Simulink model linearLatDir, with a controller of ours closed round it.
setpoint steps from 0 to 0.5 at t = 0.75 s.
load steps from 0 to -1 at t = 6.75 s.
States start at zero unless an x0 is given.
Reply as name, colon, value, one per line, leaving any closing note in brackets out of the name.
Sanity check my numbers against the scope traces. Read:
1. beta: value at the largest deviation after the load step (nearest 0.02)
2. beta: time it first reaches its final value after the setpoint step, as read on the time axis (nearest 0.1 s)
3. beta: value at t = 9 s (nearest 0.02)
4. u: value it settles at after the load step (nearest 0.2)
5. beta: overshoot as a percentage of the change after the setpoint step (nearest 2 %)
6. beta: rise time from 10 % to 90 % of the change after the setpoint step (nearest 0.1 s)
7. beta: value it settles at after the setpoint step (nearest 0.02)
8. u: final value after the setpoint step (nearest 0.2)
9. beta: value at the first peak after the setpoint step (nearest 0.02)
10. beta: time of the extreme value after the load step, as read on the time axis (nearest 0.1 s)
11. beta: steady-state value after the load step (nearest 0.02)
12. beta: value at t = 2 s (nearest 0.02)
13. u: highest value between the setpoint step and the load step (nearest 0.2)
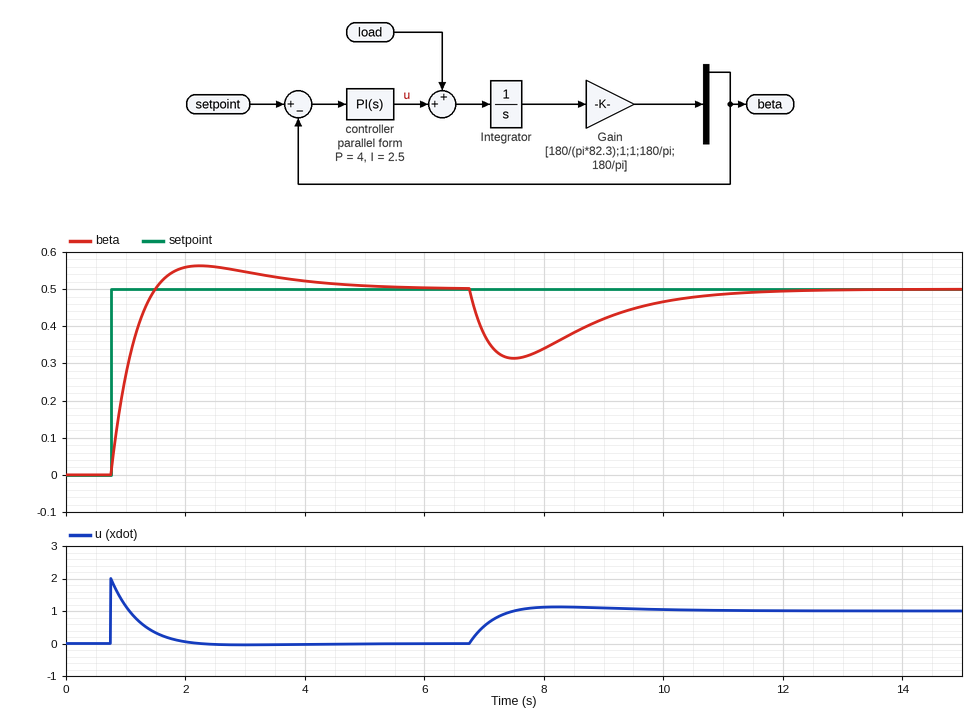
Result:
beta: value at the largest deviation after the load step: 0.32
beta: time it first reaches its final value after the setpoint step, as read on the time axis: 1.5 s
beta: value at t = 9 s: 0.42
u: value it settles at after the load step: 1.0
beta: overshoot as a percentage of the change after the setpoint step: 12 %
beta: rise time from 10 % to 90 % of the change after the setpoint step: 0.5 s
beta: value it settles at after the setpoint step: 0.50
u: final value after the setpoint step: 0.0
beta: value at the first peak after the setpoint step: 0.56
beta: time of the extreme value after the load step, as read on the time axis: 7.5 s
beta: steady-state value after the load step: 0.50
beta: value at t = 2 s: 0.56
u: highest value between the setpoint step and the load step: 2.0
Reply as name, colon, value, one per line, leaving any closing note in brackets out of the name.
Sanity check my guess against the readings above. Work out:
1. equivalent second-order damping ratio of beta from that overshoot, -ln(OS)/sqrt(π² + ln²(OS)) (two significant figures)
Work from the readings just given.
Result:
equivalent second-order damping ratio of beta from that overshoot, -ln(OS)/sqrt(π² + ln²(OS)): 0.56
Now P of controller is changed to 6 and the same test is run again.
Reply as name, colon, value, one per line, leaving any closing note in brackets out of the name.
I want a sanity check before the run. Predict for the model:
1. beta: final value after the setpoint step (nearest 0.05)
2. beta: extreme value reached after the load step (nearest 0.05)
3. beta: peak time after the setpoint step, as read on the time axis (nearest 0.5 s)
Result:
beta: final value after the setpoint step: 0.50
beta: extreme value reached after the load step: 0.35
beta: peak time after the setpoint step, as read on the time axis: 2.0 s
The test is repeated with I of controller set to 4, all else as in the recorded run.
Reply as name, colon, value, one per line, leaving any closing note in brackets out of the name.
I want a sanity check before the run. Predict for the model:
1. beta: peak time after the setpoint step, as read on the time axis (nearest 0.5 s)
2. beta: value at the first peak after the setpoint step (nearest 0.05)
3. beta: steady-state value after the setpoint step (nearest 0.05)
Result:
beta: peak time after the setpoint step, as read on the time axis: 2.0 s
beta: value at the first peak after the setpoint step: 0.60
beta: steady-state value after the setpoint step: 0.50
